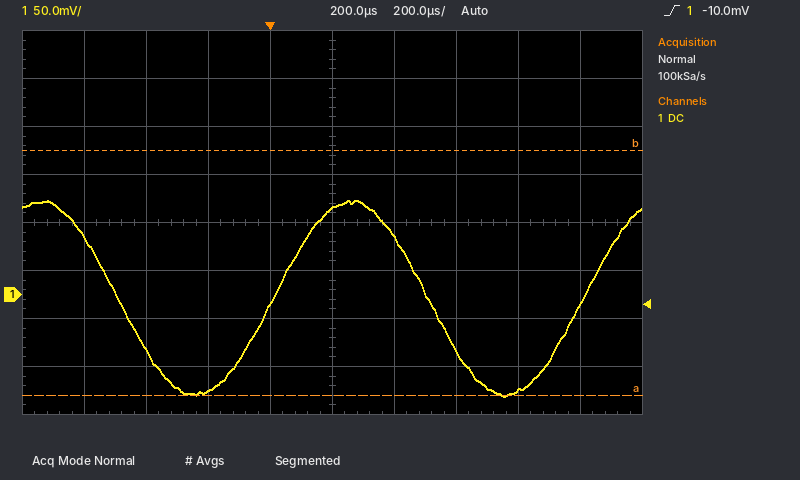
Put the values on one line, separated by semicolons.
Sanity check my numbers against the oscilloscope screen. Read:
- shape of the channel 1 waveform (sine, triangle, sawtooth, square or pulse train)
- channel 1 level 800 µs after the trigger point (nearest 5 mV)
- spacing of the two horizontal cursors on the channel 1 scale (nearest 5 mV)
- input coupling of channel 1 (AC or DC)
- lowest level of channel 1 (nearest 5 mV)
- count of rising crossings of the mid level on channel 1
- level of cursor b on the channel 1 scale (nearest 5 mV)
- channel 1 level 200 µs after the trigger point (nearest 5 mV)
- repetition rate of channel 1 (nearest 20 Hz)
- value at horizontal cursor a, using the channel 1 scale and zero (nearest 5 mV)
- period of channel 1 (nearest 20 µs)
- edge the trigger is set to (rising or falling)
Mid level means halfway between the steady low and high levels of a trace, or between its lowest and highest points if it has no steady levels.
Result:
sine; -100 mV; 255 mV; DC; -105 mV; 2; 150 mV; 90 mV; 1.00 kHz; -105 mV; 1.00 ms; rising
